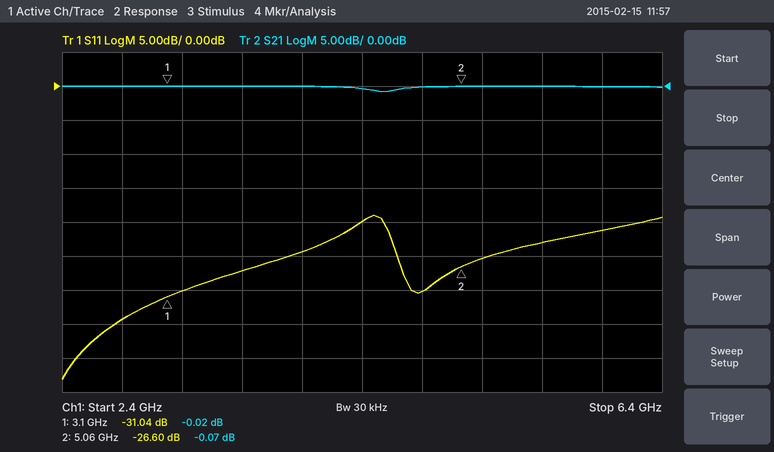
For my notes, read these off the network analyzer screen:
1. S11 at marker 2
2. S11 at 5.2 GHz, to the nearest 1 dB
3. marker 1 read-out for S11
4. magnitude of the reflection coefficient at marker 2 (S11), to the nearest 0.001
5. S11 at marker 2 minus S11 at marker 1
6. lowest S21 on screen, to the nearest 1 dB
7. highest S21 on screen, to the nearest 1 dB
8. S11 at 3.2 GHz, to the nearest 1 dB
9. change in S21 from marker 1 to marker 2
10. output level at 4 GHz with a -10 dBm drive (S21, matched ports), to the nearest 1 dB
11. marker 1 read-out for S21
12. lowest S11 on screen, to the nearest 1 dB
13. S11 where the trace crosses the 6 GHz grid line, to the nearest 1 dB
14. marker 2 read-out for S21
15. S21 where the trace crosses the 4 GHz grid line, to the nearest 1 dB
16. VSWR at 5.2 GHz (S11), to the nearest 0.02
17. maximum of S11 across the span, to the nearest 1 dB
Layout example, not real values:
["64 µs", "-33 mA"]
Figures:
["-26.60 dB", "-25 dB", "-31.04 dB", "0.047", "4.44 dB", "-1 dB", "0 dB", "-30 dB", "-0.05 dB", "-10 dBm", "-0.02 dB", "-43 dB", "-21 dB", "-0.07 dB", "0 dB", "1.12", "-19 dB"]
